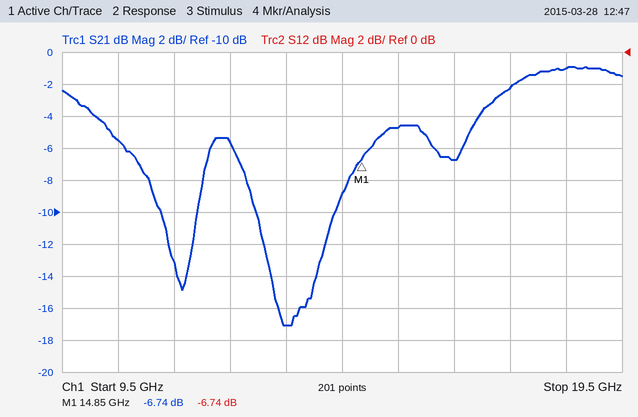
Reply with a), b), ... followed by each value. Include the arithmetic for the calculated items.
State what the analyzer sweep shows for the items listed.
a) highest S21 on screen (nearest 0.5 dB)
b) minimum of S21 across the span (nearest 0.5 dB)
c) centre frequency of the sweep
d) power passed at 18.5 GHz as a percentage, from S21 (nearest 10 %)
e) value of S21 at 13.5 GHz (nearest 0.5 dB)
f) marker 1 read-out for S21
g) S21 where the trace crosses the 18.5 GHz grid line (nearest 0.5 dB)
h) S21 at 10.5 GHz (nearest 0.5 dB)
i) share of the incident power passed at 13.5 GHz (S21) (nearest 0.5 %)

a) -1.0 dB
b) -17.0 dB
c) 14.5 GHz
d) 10^(-1/10) ≈ 79.4 %, so 80 % to the nearest 10 %
e) -17.0 dB
f) -6.74 dB
g) -1.0 dB
h) -5.5 dB
i) 10^(-17/10) ≈ 2.0 %
